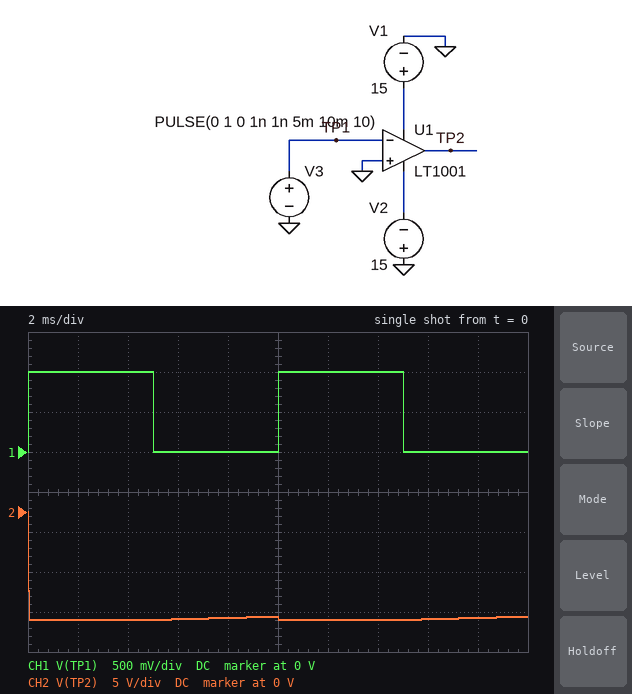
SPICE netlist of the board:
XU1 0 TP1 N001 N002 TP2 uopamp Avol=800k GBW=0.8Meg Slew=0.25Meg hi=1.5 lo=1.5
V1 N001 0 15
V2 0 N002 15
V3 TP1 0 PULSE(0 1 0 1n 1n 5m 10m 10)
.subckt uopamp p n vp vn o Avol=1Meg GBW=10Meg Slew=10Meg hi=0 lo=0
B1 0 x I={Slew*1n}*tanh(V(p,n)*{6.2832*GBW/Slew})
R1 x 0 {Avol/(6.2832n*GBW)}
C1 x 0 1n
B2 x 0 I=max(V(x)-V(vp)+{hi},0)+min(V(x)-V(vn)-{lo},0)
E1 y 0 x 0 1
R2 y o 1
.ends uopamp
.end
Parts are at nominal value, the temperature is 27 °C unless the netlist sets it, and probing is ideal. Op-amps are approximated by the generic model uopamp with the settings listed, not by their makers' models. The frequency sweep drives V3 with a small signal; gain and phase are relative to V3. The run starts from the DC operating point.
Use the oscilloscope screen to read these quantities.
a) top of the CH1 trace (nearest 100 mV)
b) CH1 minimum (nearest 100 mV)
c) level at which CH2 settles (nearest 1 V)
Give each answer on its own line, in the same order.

1.0 V
0 V
-13 V
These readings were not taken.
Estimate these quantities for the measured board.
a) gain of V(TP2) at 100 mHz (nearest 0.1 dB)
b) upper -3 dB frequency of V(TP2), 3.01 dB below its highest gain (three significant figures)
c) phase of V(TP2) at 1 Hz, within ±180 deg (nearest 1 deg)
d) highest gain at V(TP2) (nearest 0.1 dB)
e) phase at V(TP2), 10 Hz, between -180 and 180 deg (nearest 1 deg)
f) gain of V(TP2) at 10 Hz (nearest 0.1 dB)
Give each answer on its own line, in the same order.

118.0 dB
1.00 Hz
135 deg
118.1 dB
96 deg
98.0 dB
